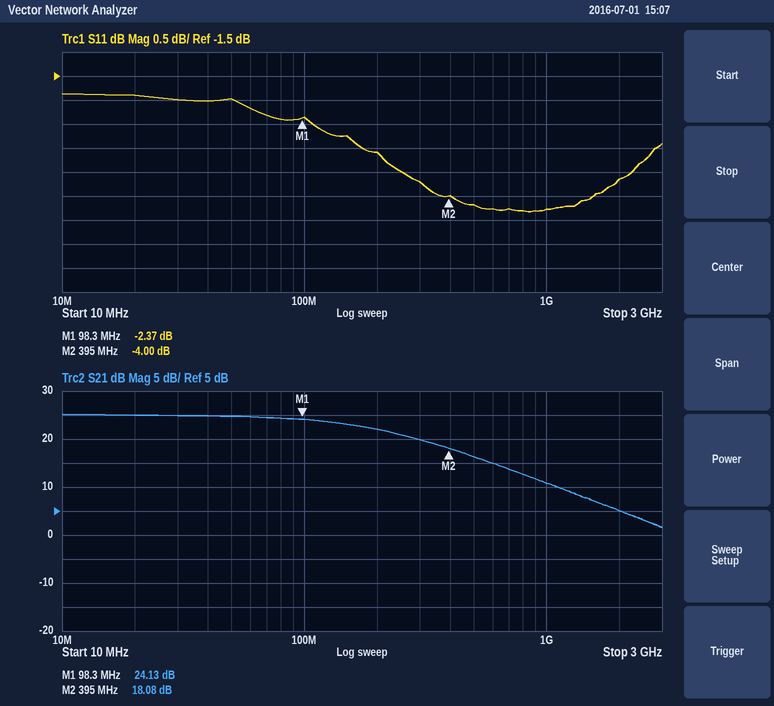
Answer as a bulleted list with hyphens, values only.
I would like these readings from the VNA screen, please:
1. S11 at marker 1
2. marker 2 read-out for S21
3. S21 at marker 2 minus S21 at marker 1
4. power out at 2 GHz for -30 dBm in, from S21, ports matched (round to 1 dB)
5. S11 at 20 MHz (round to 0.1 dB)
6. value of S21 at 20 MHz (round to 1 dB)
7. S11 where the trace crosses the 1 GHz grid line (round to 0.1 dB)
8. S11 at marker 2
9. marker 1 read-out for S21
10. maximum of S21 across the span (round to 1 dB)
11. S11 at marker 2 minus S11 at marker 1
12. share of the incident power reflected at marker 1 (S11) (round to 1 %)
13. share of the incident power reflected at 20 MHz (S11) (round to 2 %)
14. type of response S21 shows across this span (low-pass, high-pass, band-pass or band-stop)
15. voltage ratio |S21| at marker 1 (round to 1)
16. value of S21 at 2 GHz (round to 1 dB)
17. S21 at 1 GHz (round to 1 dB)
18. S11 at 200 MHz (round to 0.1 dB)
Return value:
- -2.37 dB
- 18.08 dB
- -6.05 dB
- -25 dBm
- -1.9 dB
- 25 dB
- -4.3 dB
- -4.00 dB
- 24.13 dB
- 25 dB
- -1.63 dB
- 58 %
- 64 %
- low-pass
- 16
- 5 dB
- 11 dB
- -3.1 dB
